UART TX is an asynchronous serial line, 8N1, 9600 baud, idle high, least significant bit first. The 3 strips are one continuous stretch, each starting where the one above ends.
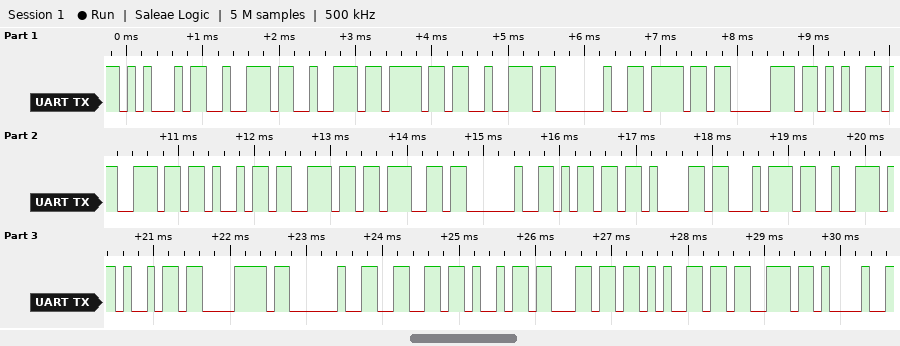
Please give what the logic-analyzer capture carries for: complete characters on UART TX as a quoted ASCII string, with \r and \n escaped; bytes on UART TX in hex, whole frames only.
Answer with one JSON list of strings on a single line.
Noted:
["\"Error opening matrix files!\"", "45 72 72 6F 72 20 6F 70 65 6E 69 6E 67 20 6D 61 74 72 69 78 20 66 69 6C 65 73 21"]
